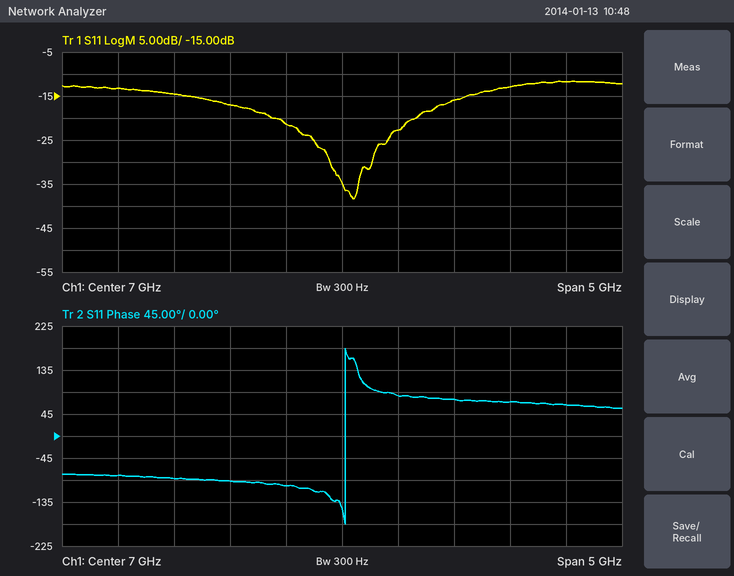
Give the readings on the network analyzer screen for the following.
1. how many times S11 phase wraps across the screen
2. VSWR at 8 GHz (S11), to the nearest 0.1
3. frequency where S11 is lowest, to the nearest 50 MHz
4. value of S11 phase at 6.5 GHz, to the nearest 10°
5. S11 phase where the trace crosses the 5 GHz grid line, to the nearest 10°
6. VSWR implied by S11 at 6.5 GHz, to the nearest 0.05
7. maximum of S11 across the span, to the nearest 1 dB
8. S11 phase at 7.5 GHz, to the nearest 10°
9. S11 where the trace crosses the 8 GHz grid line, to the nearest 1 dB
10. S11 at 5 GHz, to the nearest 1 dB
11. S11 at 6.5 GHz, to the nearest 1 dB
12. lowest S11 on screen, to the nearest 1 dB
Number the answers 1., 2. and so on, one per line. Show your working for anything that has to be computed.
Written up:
1. 1
2. |Γ| = 10^(-16/20) = 0.1585; VSWR = (1 + 0.1585)/(1 − 0.1585) ≈ 1.4
3. 7.10 GHz
4. -100°
5. -80°
6. |Γ| = 10^(-21/20) = 0.0891; VSWR = (1 + 0.0891)/(1 − 0.0891) ≈ 1.20
7. -12 dB
8. 80°
9. -16 dB
10. -13 dB
11. -21 dB
12. -38 dB
